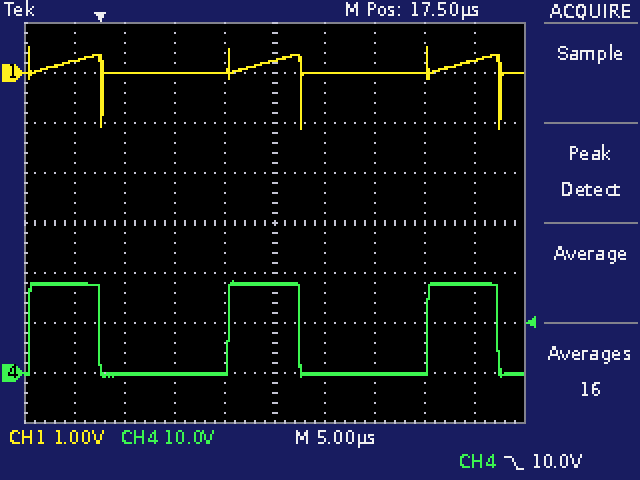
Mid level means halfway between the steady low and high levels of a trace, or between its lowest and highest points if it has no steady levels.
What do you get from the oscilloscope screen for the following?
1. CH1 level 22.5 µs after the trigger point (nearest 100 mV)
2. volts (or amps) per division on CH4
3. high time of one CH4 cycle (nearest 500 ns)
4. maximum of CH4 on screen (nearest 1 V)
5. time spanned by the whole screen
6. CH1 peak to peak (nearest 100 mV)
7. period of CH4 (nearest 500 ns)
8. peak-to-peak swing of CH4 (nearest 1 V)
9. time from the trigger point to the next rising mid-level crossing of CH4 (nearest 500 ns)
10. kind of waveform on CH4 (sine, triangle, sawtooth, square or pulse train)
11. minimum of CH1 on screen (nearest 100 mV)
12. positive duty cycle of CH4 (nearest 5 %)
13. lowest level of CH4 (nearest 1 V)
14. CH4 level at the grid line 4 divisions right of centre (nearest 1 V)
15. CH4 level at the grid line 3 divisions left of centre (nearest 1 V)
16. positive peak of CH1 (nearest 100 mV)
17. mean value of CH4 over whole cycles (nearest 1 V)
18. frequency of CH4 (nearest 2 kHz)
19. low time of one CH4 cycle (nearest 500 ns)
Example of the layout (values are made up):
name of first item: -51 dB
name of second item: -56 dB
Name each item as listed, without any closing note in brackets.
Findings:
CH1 level 22.5 µs after the trigger point: 0.0 V
volts (or amps) per division on CH4: 10 V
high time of one CH4 cycle: 7.0 µs
maximum of CH4 on screen: 18 V
time spanned by the whole screen: 50 µs
CH1 peak to peak: 1.6 V
period of CH4: 20.0 µs
peak-to-peak swing of CH4: 19 V
time from the trigger point to the next rising mid-level crossing of CH4: 13.0 µs
kind of waveform on CH4: pulse train
minimum of CH1 on screen: -1.1 V
positive duty cycle of CH4: 35 %
lowest level of CH4: -1 V
CH4 level at the grid line 4 divisions right of centre: 18 V
CH4 level at the grid line 3 divisions left of centre: 0 V
positive peak of CH1: 500 mV
mean value of CH4 over whole cycles: 6 V
frequency of CH4: 50 kHz
low time of one CH4 cycle: 13.0 µs
